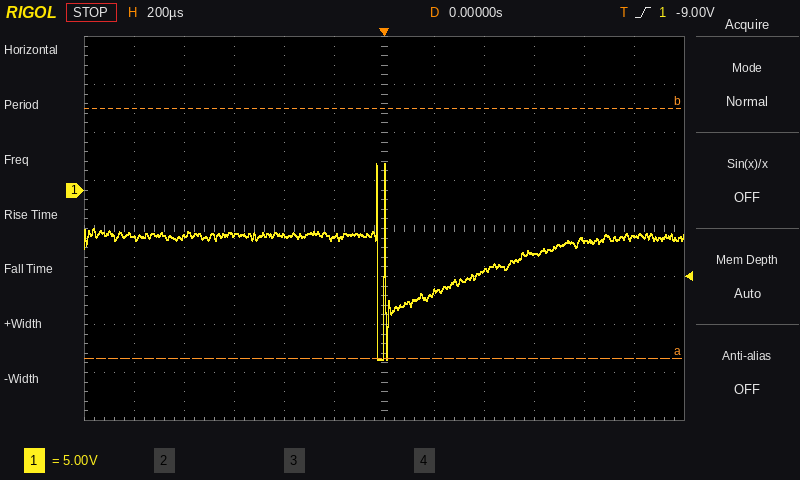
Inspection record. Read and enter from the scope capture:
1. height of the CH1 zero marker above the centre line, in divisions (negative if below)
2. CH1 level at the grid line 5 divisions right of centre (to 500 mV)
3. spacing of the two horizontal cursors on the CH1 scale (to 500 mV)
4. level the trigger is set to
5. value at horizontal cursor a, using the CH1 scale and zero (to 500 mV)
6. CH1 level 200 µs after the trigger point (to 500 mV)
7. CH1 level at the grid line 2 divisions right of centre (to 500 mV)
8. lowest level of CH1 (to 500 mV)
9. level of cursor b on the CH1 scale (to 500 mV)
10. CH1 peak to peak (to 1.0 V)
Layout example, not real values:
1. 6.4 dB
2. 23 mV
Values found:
1. +0.8 div
2. -5.0 V
3. 26.0 V
4. -9.00 V
5. -17.5 V
6. -10.5 V
7. -8.5 V
8. -17.5 V
9. 8.5 V
10. 20.0 V
